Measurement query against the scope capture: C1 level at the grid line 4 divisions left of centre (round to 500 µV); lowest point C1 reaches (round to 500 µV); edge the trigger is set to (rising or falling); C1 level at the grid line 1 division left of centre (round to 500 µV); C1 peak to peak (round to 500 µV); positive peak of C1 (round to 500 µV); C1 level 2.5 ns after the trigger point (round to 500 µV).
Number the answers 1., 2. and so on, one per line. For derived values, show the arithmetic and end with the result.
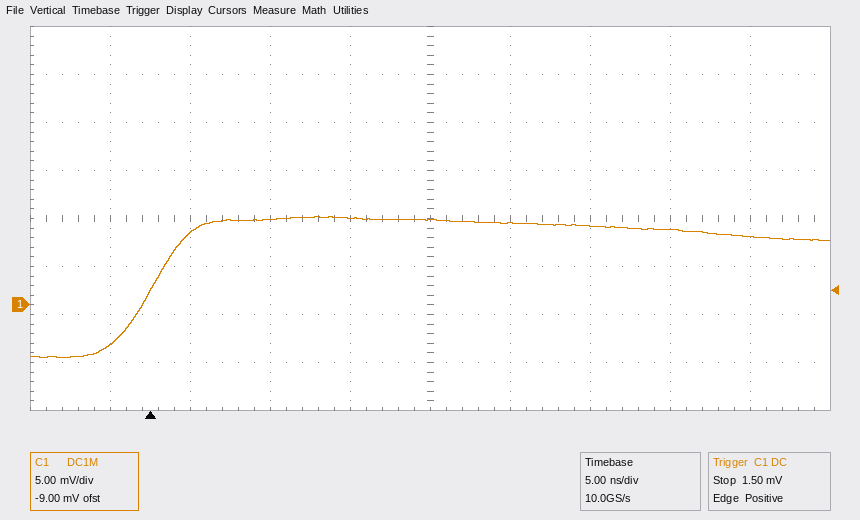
1. -4.0 mV
2. -5.5 mV
3. rising
4. 9.0 mV
5. 9.0 mV − (-5.5 mV) = 14.5 mV
6. 9.0 mV
7. 7.5 mV
